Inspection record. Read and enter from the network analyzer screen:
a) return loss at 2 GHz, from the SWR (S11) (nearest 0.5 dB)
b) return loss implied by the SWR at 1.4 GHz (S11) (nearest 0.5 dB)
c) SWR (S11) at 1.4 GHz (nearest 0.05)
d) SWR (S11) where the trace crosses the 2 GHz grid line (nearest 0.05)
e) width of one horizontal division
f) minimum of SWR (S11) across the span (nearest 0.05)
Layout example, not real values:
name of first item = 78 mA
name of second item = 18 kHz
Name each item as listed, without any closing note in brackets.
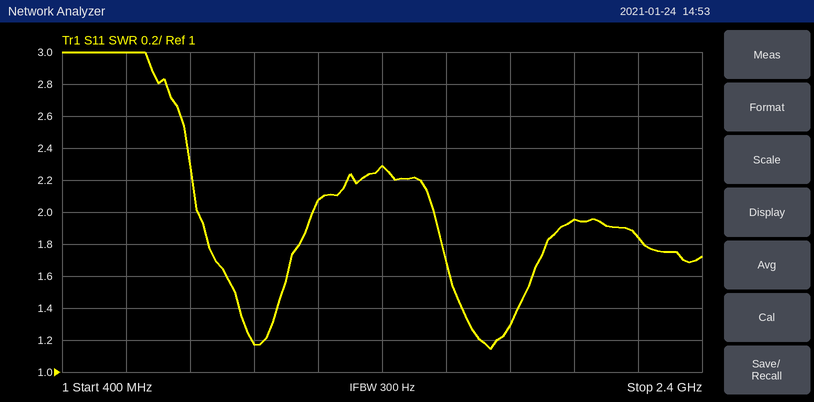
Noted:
return loss at 2 GHz, from the SWR (S11) = 10.0 dB
return loss implied by the SWR at 1.4 GHz (S11) = 8.0 dB
SWR (S11) at 1.4 GHz = 2.30
SWR (S11) where the trace crosses the 2 GHz grid line = 1.95
width of one horizontal division = 200 MHz
minimum of SWR (S11) across the span = 1.15
